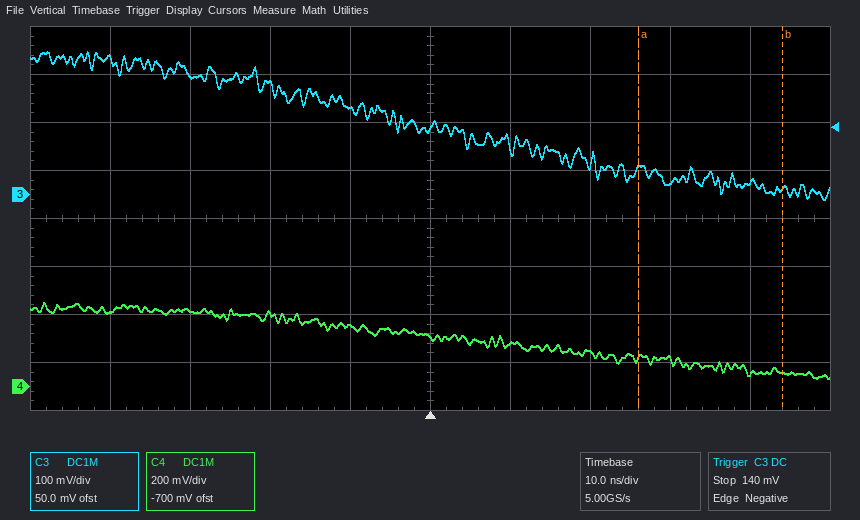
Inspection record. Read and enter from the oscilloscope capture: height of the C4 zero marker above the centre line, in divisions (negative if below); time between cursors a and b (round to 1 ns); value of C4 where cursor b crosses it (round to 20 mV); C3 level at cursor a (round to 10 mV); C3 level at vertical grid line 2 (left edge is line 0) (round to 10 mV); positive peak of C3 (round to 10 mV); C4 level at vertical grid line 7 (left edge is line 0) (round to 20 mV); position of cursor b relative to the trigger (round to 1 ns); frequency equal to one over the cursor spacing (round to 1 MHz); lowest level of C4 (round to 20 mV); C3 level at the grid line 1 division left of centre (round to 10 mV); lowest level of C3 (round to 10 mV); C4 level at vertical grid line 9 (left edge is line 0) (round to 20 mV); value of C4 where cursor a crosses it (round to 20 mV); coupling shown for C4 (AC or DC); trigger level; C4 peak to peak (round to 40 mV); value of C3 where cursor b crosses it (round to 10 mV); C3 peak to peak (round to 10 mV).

-3.5 div
18 ns
60 mV
50 mV
250 mV
300 mV
140 mV
+44 ns
56 MHz
40 mV
180 mV
-10 mV
60 mV
120 mV
DC
140 mV
320 mV
10 mV
310 mV
